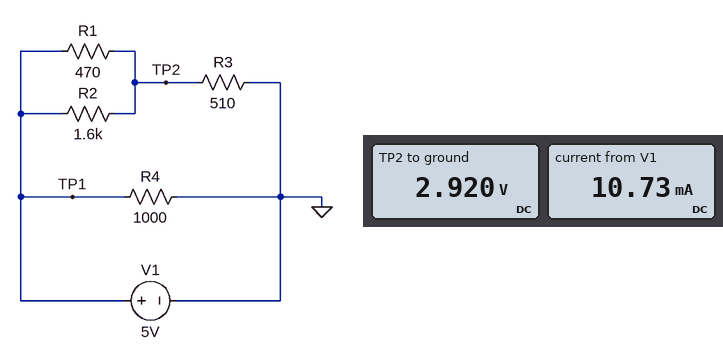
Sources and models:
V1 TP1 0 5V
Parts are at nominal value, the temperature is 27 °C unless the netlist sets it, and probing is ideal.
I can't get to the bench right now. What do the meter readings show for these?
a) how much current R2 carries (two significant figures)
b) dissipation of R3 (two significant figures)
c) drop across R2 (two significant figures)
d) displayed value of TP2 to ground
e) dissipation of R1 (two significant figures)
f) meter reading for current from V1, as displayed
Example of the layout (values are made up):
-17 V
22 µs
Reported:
1.3 mA
17 mW
2.1 V
2.920 V
9.2 mW
10.73 mA
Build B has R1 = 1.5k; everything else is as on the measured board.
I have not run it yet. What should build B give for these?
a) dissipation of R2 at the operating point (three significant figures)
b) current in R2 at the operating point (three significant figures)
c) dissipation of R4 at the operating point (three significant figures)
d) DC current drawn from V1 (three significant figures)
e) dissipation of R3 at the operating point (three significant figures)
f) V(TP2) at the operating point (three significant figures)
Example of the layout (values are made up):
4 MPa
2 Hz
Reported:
5.68 mW
1.88 mA
25.0 mW
8.89 mA
7.73 mW
1.99 V
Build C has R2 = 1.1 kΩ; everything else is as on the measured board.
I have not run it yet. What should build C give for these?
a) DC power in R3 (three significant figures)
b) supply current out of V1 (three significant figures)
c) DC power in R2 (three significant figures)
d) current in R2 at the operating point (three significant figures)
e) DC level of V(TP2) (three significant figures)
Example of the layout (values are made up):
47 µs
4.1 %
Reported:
18.1 mW
11.0 mA
3.50 mW
1.78 mA
3.04 V
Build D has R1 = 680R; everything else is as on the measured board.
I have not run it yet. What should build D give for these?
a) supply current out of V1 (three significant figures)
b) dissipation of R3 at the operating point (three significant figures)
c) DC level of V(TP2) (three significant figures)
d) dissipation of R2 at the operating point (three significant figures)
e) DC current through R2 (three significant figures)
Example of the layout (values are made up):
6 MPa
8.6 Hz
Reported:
10.1 mA
13.1 mW
2.58 V
3.65 mW
1.51 mA
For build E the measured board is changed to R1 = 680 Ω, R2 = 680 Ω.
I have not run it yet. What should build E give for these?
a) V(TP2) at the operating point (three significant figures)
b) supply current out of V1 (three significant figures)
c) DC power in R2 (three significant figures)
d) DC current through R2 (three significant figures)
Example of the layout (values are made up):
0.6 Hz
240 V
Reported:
3.00 V
10.9 mA
5.88 mW
2.94 mA
